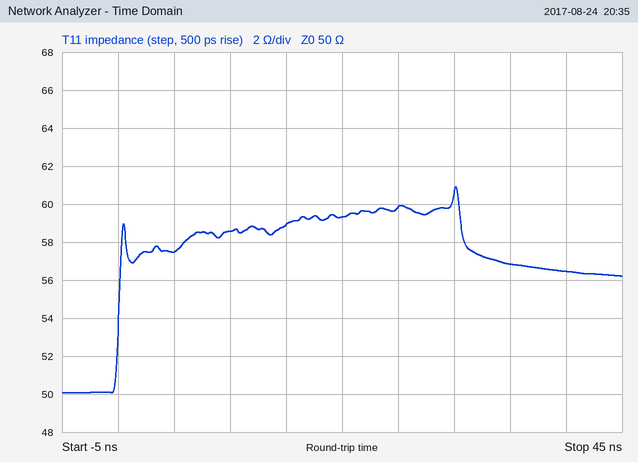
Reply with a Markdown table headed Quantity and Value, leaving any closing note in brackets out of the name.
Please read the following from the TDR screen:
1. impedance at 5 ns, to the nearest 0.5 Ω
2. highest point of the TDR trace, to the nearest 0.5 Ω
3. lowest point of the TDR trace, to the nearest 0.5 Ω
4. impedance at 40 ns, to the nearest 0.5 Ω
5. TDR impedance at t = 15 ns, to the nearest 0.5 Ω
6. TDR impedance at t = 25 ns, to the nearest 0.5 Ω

| Quantity | Value |
|---|---|
| impedance at 5 ns, to the nearest 0.5 Ω | 57.5 Ω |
| highest point of the TDR trace, to the nearest 0.5 Ω | 61.0 Ω |
| lowest point of the TDR trace, to the nearest 0.5 Ω | 50.0 Ω |
| impedance at 40 ns, to the nearest 0.5 Ω | 56.5 Ω |
| TDR impedance at t = 15 ns, to the nearest 0.5 Ω | 59.0 Ω |
| TDR impedance at t = 25 ns, to the nearest 0.5 Ω | 60.0 Ω |
